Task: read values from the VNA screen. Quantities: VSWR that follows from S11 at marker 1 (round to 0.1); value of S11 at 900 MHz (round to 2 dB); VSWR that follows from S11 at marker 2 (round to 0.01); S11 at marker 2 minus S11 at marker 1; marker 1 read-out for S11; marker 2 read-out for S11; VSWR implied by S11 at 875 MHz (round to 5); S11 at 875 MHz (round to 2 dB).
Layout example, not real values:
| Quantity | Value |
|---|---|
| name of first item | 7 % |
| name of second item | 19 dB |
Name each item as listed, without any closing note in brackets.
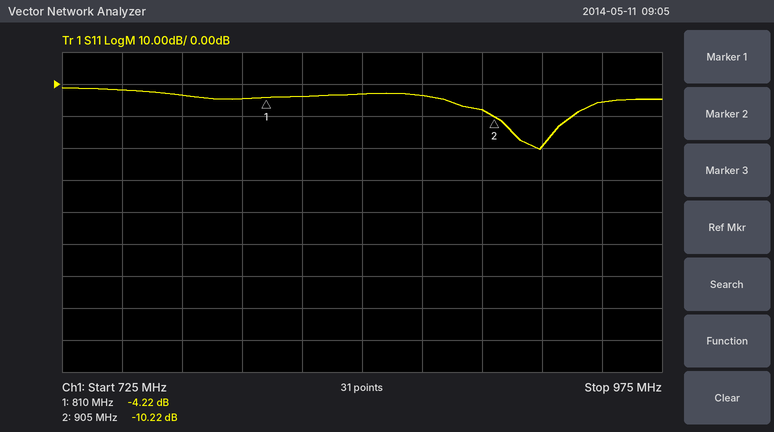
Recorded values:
| Quantity | Value |
|---|---|
| VSWR that follows from S11 at marker 1 | 4.2 |
| value of S11 at 900 MHz | -8 dB |
| VSWR that follows from S11 at marker 2 | 1.89 |
| S11 at marker 2 minus S11 at marker 1 | -6.00 dB |
| marker 1 read-out for S11 | -4.22 dB |
| marker 2 read-out for S11 | -10.22 dB |
| VSWR implied by S11 at 875 MHz | 5 |
| S11 at 875 MHz | -4 dB |
